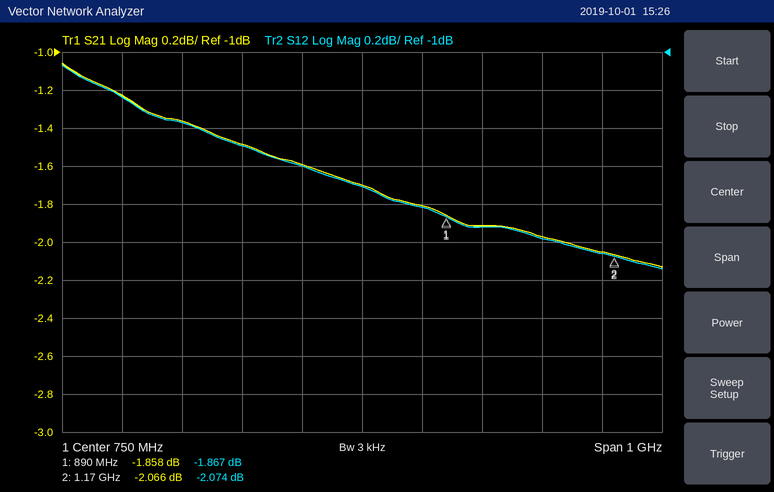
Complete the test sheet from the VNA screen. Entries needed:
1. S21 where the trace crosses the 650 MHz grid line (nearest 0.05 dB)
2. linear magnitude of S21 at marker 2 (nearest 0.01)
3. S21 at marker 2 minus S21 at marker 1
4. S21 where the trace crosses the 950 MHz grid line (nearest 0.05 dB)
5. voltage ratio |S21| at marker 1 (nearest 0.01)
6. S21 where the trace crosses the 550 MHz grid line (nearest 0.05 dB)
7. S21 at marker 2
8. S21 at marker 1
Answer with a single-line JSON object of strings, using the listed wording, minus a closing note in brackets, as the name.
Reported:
{"S21 where the trace crosses the 650 MHz grid line": "-1.60 dB", "linear magnitude of S21 at marker 2": "0.79", "S21 at marker 2 minus S21 at marker 1": "-0.208 dB", "S21 where the trace crosses the 950 MHz grid line": "-1.90 dB", "voltage ratio |S21| at marker 1": "0.81", "S21 where the trace crosses the 550 MHz grid line": "-1.50 dB", "S21 at marker 2": "-2.066 dB", "S21 at marker 1": "-1.858 dB"}
